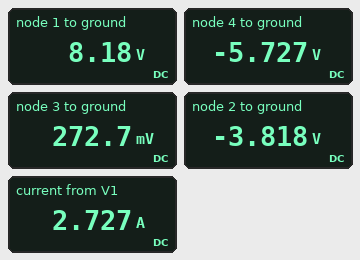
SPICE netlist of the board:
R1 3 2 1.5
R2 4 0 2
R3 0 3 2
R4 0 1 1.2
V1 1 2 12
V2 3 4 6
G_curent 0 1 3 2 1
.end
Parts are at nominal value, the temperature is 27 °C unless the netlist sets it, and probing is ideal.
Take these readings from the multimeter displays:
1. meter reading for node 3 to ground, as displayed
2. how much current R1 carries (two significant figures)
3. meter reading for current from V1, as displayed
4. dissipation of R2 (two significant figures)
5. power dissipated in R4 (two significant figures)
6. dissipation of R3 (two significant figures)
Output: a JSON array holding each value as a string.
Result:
["272.7 mV", "2.7 A", "2.727 A", "16 W", "56 W", "37 mW"]
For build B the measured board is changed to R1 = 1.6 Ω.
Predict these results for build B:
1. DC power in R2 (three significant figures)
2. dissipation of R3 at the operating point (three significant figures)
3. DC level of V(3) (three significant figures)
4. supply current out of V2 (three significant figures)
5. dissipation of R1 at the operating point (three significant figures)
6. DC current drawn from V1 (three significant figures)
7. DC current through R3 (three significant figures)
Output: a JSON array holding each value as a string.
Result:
["15.8 W", "71.3 mW", "378 mV", "2.81 A", "11.0 W", "2.62 A", "189 mA"]
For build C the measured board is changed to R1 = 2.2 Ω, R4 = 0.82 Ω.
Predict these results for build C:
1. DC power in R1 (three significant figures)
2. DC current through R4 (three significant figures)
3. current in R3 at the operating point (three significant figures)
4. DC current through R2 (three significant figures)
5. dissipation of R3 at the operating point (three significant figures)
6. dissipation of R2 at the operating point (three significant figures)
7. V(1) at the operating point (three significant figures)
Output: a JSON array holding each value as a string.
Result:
["14.6 W", "8.24 A", "212 mA", "2.79 A", "90.1 mW", "15.5 W", "6.76 V"]
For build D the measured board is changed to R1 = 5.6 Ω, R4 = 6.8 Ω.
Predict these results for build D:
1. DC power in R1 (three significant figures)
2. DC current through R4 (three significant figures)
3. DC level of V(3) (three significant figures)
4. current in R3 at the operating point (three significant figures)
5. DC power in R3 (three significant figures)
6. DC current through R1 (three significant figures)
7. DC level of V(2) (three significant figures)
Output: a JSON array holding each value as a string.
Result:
["475 mW", "1.92 A", "2.71 V", "1.35 A", "3.67 W", "291 mA", "1.08 V"]
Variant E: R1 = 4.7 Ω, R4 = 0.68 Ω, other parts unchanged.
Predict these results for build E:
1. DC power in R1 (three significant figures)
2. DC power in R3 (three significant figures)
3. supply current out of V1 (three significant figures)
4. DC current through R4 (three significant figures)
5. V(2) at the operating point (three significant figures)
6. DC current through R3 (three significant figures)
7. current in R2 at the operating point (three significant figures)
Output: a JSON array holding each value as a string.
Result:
["11.5 W", "1.03 W", "1.57 A", "8.93 A", "-5.93 V", "717 mA", "2.28 A"]
